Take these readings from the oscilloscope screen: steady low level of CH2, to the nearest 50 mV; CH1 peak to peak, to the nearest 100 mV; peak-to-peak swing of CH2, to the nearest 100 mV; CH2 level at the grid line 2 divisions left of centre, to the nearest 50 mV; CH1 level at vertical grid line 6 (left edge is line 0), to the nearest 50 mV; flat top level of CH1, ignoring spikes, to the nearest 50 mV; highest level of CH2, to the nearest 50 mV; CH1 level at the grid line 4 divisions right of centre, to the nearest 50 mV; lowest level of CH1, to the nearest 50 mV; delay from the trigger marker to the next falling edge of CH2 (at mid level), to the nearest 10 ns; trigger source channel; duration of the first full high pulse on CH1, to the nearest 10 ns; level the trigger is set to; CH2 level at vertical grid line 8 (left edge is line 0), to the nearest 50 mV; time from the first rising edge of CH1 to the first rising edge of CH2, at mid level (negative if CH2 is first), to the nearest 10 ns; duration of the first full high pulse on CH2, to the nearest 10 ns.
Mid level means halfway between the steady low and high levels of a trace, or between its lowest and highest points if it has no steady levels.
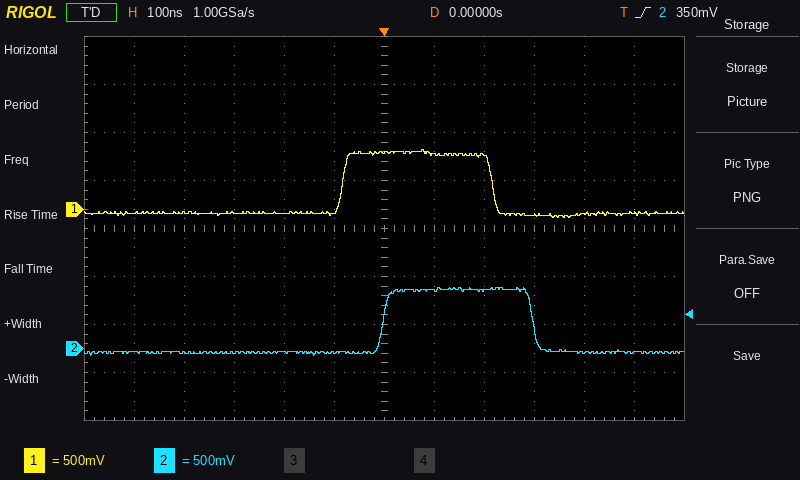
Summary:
-50 mV
700 mV
700 mV
-50 mV
600 mV
600 mV
650 mV
-50 mV
-100 mV
300 ns
CH2
300 ns
350 mV
600 mV
+80 ns
300 ns
